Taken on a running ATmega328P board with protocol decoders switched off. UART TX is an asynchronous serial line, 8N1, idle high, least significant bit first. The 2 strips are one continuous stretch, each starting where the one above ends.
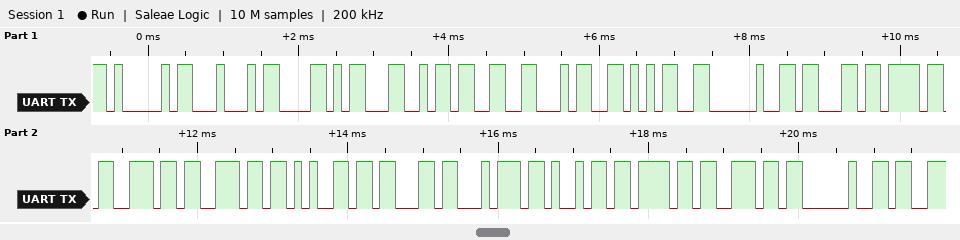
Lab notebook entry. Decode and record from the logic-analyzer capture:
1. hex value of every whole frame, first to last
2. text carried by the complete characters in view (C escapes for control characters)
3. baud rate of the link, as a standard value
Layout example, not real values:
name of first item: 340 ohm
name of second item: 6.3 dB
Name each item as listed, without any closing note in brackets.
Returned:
hex value of every whole frame, first to last: 41 44 58 4C 33 34 35 20 63 6F 6E 6E 65 63 74 69 6F 6E 20
text carried by the complete characters in view: "ADXL345 connection "
baud rate of the link, as a standard value: 9600 baud
